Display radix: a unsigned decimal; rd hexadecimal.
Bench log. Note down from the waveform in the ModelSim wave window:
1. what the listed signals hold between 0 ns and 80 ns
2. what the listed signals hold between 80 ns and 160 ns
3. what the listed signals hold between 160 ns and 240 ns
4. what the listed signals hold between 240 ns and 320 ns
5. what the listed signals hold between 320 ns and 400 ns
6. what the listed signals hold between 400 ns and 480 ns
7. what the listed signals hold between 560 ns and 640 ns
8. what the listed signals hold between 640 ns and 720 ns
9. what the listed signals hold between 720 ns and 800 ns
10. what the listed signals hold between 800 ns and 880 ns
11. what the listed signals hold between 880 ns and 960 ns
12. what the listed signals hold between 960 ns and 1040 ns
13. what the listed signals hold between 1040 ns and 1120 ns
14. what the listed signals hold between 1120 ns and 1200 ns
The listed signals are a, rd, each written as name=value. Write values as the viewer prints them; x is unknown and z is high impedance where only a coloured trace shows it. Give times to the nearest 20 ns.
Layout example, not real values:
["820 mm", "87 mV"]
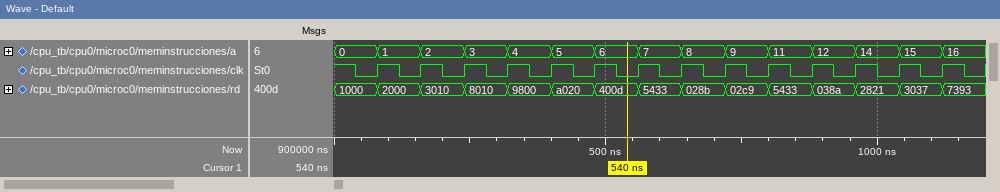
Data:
["a=0, rd=1000", "a=1, rd=2000", "a=2, rd=3010", "a=3, rd=8010", "a=4, rd=9800", "a=5, rd=a020", "a=7, rd=5433", "a=8, rd=028b", "a=9, rd=02c9", "a=11, rd=5433", "a=12, rd=038a", "a=14, rd=2821", "a=15, rd=3037", "a=16, rd=7393"]
